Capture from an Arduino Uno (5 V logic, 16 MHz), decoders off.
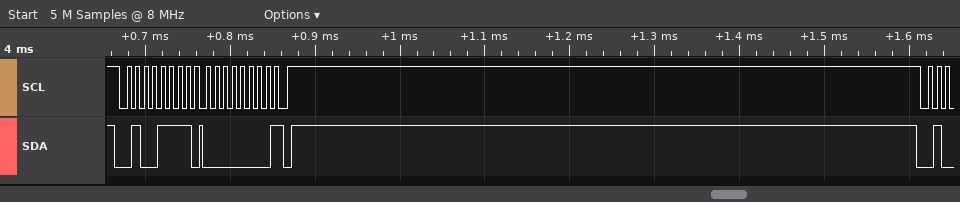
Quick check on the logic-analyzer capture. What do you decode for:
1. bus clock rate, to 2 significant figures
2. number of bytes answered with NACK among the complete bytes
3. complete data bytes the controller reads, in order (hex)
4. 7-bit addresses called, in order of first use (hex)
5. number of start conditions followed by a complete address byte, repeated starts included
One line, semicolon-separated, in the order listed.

100 kHz; 1; 00; 0x27; 1
